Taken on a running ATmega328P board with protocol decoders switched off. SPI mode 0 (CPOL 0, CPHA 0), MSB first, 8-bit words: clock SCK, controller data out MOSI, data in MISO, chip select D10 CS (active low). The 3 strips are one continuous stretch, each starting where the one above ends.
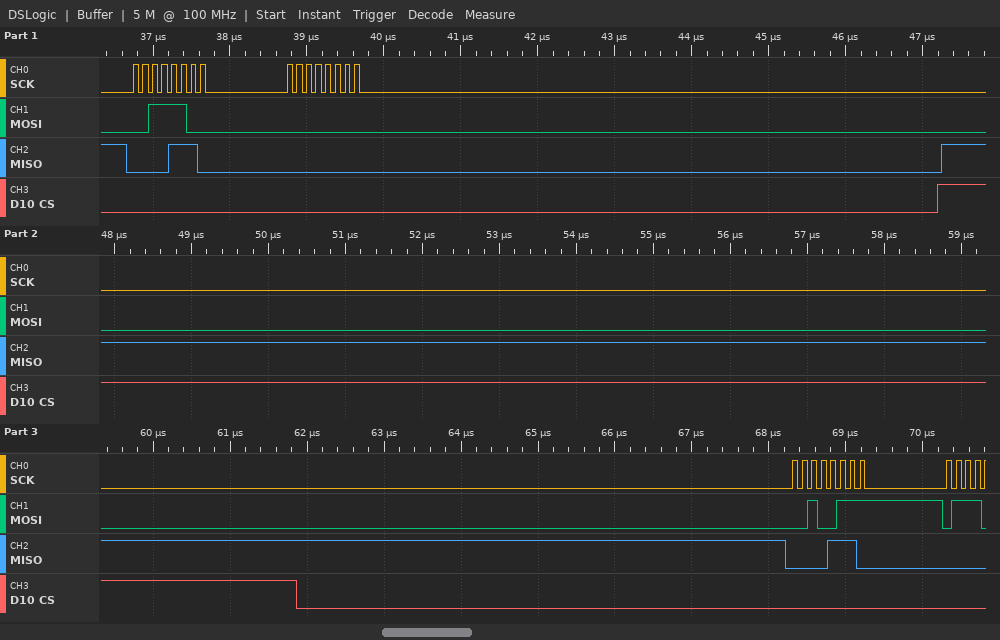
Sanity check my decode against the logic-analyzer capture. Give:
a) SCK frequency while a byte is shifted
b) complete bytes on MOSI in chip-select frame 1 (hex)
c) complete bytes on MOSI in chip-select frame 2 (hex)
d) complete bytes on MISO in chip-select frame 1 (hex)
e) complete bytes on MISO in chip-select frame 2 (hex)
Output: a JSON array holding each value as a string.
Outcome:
["8 MHz", "0x3C 0x00", "0x27", "0x0E 0x00", "0x0E"]
